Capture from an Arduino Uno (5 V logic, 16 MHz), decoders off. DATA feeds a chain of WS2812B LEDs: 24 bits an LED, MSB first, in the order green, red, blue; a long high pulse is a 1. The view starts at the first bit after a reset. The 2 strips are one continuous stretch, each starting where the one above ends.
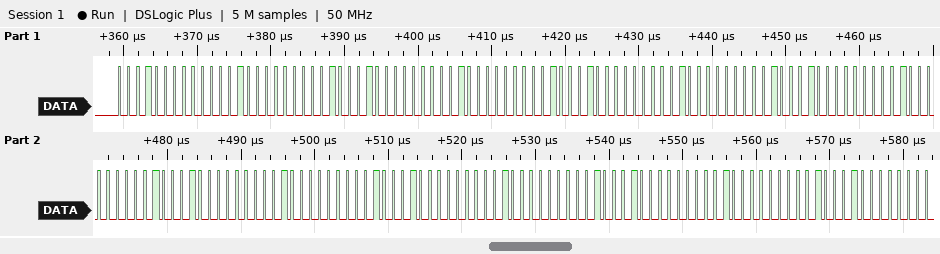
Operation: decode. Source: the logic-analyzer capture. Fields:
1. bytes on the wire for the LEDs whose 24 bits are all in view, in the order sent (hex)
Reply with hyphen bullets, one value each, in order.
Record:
- 10 04 01 10 04 01 10 04 01 10 04 01 10 04 01 10 04 01 10 04 01
